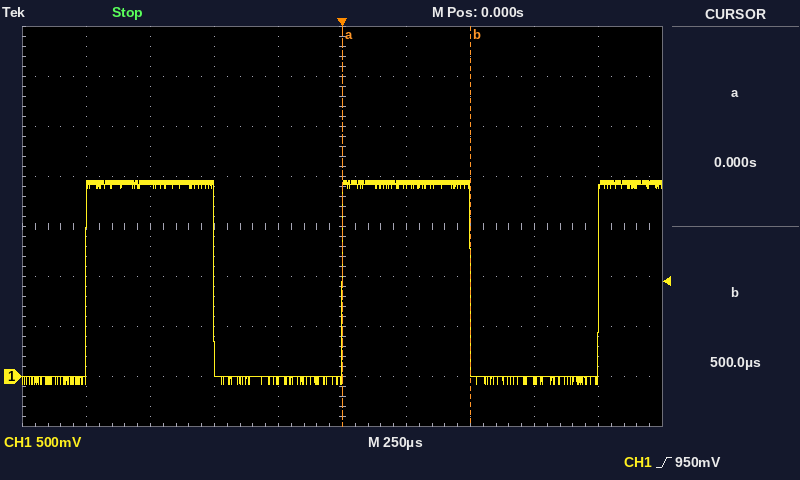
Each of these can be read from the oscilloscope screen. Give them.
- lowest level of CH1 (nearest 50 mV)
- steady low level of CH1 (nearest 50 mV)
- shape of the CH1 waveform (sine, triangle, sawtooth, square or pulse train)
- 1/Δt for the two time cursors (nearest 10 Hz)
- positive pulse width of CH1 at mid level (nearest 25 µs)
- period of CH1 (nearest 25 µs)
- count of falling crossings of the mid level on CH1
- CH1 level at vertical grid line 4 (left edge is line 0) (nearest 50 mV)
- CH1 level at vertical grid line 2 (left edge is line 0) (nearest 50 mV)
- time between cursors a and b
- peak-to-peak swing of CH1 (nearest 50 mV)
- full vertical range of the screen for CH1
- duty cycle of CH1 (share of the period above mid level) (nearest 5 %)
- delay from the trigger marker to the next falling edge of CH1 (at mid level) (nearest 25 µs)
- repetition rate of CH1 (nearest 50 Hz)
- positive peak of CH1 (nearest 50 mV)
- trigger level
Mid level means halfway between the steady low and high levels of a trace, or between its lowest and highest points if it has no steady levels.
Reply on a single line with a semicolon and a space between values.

-100 mV; 0 mV; square; 2.00 kHz; 500 µs; 1.000 ms; 2; -50 mV; 1.95 V; 500 µs; 2.05 V; 4 V; 50 %; 500 µs; 1.00 kHz; 1.95 V; 950 mV
